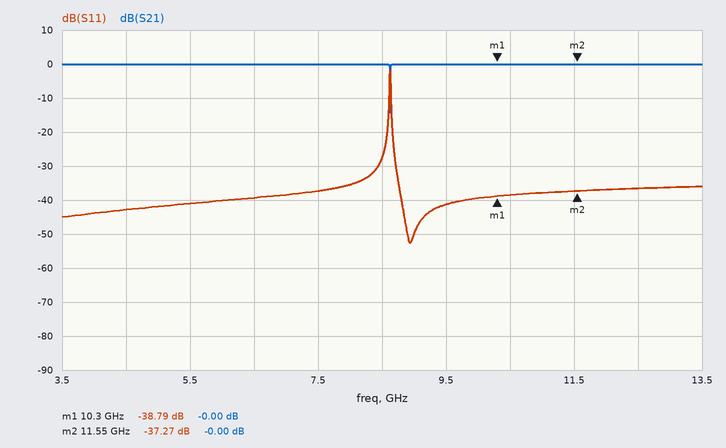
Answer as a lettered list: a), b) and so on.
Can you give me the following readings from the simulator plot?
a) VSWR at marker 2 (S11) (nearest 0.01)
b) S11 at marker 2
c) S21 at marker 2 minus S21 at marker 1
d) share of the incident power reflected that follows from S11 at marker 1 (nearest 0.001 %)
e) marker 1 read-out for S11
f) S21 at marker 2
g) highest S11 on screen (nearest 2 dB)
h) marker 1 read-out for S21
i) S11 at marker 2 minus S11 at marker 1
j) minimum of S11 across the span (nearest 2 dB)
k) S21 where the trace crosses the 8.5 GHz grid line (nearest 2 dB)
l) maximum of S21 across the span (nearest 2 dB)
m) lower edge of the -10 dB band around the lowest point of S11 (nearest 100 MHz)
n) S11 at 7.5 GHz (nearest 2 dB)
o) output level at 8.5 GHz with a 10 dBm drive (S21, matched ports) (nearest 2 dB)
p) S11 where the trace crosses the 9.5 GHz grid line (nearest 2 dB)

a) 1.03
b) -37.27 dB
c) 0.00 dB
d) 0.013 %
e) -38.79 dB
f) -0.00 dB
g) -2 dB
h) -0.00 dB
i) 1.52 dB
j) -52 dB
k) 0 dB
l) 0 dB
m) 8.6 GHz
n) -38 dB
o) 10 dBm
p) -42 dB
